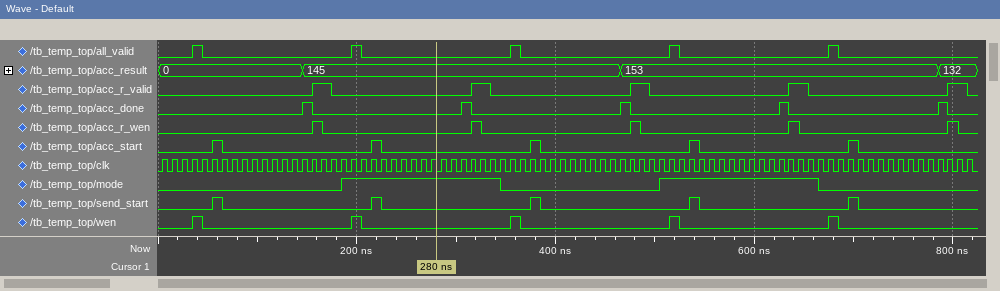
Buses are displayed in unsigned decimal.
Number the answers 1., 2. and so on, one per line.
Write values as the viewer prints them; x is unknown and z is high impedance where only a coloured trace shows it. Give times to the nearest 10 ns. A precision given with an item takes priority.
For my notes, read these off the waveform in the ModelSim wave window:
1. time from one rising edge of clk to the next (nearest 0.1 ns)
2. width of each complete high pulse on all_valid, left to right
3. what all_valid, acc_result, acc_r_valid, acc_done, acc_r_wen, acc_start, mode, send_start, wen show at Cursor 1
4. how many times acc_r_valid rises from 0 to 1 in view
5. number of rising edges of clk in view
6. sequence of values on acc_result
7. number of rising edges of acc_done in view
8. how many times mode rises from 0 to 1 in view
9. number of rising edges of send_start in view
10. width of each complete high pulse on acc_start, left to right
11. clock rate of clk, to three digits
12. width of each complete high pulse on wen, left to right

1. 10 ns
2. 10 ns, 10 ns, 10 ns, 10 ns, 10 ns
3. all_valid=0, acc_result=145, acc_r_valid=0, acc_done=0, acc_r_wen=0, acc_start=0, mode=1, send_start=0, wen=0
4. 5
5. 82
6. 0, 145, 153, 132
7. 5
8. 2
9. 5
10. 10 ns, 10 ns, 10 ns, 10 ns, 10 ns
11. 100 MHz
12. 10 ns, 10 ns, 10 ns, 10 ns, 10 ns
